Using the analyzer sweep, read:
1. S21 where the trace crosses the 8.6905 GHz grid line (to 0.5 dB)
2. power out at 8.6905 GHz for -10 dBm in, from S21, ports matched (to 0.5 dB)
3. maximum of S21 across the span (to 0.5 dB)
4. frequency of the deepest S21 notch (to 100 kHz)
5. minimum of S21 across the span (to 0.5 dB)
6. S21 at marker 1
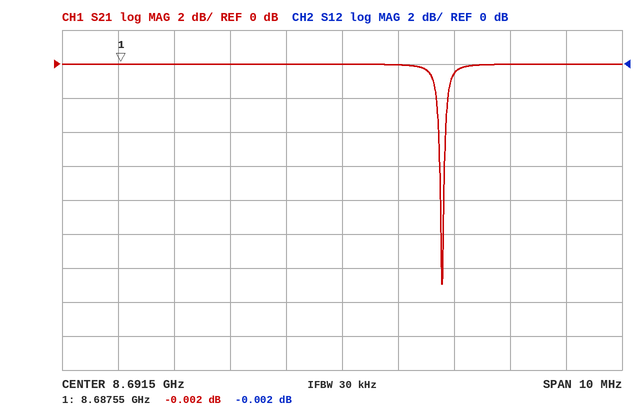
0.0 dB
-10.0 dBm
0.0 dB
8.6933 GHz
-13.0 dB
-0.002 dB
